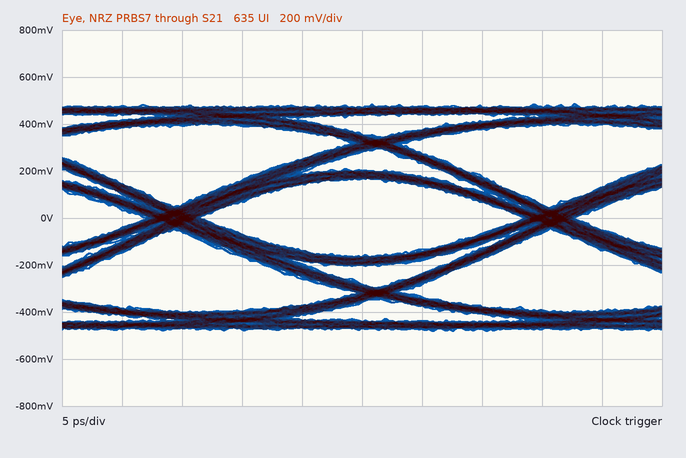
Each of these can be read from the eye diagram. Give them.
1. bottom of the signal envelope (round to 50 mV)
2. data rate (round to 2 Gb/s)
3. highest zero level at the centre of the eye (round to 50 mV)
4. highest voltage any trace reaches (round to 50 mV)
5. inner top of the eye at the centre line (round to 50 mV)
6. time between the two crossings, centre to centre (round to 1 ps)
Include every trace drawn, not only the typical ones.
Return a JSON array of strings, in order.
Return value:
["-500 mV", "32 Gb/s", "-150 mV", "500 mV", "150 mV", "31 ps"]
